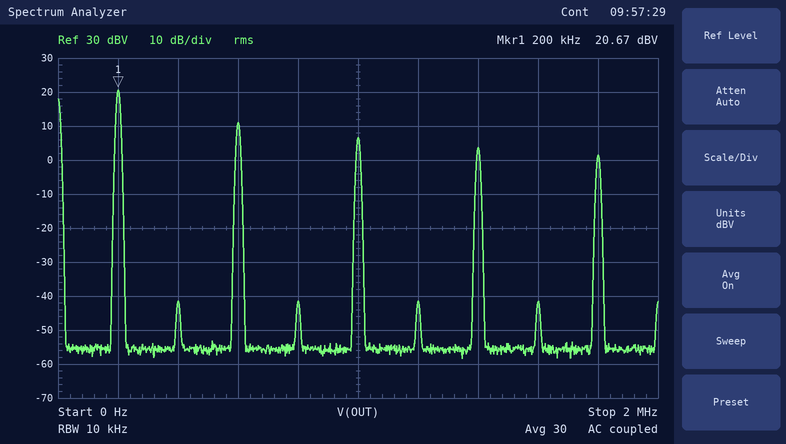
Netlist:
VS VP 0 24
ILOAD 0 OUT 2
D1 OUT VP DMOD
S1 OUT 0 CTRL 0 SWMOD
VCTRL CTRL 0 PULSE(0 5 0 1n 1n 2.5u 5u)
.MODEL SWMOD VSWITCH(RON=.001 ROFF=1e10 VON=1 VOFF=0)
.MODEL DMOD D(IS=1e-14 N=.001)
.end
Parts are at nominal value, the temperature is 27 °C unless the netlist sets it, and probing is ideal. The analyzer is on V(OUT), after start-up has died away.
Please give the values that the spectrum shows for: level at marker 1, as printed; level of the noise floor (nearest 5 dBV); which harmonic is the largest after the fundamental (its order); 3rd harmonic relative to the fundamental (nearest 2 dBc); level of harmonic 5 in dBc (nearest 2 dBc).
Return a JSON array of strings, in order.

["20.67 dBV", "-55 dBV", "3", "-10 dBc", "-14 dBc"]
